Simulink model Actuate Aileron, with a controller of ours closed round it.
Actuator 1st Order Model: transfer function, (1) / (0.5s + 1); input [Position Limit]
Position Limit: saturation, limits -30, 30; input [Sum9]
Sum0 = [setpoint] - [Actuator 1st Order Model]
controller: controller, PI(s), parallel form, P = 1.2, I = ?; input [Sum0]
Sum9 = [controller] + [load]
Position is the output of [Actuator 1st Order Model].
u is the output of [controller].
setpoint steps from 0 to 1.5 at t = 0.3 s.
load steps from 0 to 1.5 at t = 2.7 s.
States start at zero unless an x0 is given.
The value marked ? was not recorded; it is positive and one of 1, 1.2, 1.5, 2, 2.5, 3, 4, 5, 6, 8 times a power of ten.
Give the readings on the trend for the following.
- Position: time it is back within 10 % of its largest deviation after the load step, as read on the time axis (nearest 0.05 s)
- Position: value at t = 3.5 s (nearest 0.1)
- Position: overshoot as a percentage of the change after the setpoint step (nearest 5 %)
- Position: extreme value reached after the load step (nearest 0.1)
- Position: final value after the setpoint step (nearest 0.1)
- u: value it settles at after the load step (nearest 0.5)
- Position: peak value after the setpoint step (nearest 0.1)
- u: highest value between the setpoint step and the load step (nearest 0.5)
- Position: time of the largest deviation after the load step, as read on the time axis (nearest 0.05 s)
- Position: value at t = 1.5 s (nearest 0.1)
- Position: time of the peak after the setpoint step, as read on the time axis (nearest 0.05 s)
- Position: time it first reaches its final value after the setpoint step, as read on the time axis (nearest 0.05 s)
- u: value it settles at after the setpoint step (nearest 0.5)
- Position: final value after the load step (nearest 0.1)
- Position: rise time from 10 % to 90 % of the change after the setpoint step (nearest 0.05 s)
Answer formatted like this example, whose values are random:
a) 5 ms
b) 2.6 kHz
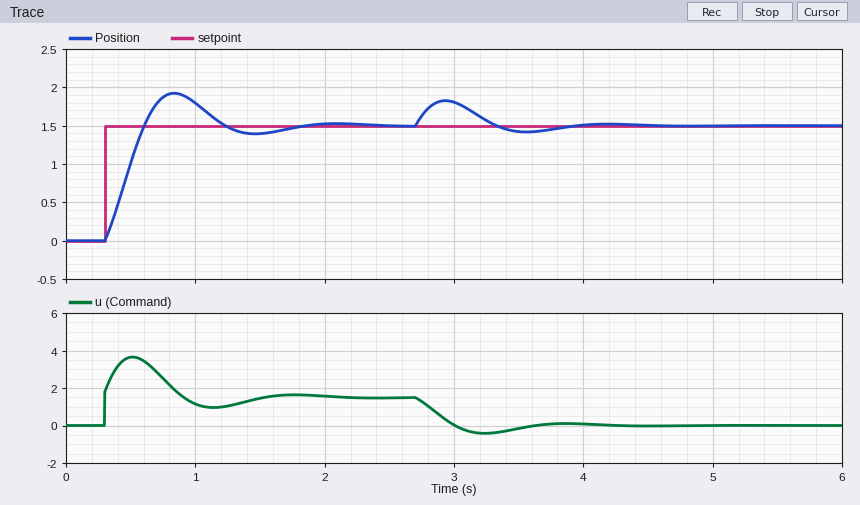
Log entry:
a) 3.80 s
b) 1.4
c) 30 %
d) 1.8
e) 1.5
f) 0.0
g) 1.9
h) 3.5
i) 2.95 s
j) 1.4
k) 0.85 s
l) 0.60 s
m) 1.5
n) 1.5
o) 0.25 s
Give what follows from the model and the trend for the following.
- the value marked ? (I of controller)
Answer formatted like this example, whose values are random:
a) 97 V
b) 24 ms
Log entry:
a) 15
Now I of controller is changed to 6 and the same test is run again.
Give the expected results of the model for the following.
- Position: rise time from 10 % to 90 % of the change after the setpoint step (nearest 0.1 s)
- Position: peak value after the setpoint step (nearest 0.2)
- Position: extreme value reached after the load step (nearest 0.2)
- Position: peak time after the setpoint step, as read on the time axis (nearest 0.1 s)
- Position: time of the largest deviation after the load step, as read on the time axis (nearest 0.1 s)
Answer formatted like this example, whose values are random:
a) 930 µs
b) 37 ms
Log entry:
a) 0.4 s
b) 1.6
c) 2.0
d) 1.2 s
e) 3.0 s
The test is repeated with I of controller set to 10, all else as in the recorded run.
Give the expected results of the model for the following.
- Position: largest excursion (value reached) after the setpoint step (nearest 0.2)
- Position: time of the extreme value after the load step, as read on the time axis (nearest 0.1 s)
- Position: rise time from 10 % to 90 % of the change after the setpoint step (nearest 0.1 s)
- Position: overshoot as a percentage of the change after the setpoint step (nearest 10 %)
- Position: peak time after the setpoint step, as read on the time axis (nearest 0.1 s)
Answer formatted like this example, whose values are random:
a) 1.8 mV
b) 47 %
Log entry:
a) 1.8
b) 3.0 s
c) 0.3 s
d) 20 %
e) 1.0 s
